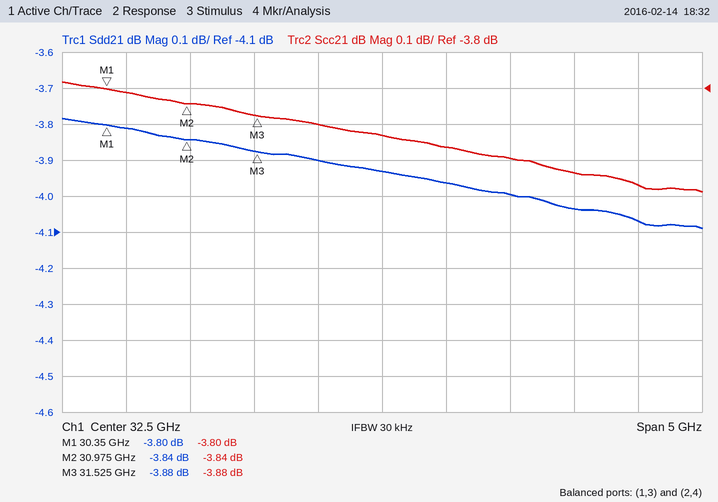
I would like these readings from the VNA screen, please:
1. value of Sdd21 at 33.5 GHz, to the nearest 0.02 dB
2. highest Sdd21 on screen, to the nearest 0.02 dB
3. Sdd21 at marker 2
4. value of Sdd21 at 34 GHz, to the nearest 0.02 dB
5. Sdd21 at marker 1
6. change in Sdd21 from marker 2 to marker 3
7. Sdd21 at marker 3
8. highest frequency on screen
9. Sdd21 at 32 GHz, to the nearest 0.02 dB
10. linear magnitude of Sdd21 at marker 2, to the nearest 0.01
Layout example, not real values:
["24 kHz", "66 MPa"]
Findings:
["-4.00 dB", "-3.78 dB", "-3.84 dB", "-4.04 dB", "-3.80 dB", "-0.04 dB", "-3.88 dB", "35 GHz", "-3.90 dB", "0.64"]
